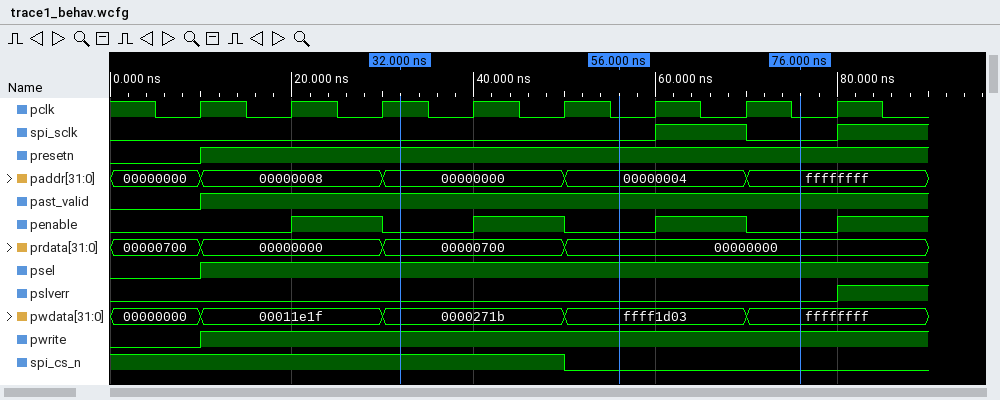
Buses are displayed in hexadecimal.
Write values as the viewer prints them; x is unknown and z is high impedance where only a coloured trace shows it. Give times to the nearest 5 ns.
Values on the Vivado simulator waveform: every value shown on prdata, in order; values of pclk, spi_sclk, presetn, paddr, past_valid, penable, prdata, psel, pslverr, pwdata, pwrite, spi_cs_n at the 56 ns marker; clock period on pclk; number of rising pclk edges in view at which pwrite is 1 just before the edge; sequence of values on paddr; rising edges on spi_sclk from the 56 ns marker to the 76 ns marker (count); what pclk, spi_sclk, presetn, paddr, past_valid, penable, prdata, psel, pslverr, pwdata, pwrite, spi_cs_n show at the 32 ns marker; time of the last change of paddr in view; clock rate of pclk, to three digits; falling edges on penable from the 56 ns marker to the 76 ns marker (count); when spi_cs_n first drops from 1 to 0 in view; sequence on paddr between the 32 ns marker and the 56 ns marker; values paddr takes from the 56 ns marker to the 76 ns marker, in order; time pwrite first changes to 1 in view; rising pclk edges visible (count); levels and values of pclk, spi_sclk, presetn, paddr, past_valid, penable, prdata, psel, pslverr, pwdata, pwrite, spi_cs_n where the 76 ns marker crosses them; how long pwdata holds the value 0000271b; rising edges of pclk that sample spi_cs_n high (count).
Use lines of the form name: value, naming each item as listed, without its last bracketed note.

every value shown on prdata, in order: 00000700, 00000000, 00000700, 00000000
values of pclk, spi_sclk, presetn, paddr, past_valid, penable, prdata, psel, pslverr, pwdata, pwrite, spi_cs_n at the 56 ns marker: pclk=0, spi_sclk=0, presetn=1, paddr=00000004, past_valid=1, penable=0, prdata=00000000, psel=1, pslverr=0, pwdata=ffff1d03, pwrite=1, spi_cs_n=0
clock period on pclk: 10 ns
number of rising pclk edges in view at which pwrite is 1 just before the edge: 7
sequence of values on paddr: 00000000, 00000008, 00000000, 00000004, ffffffff
rising edges on spi_sclk from the 56 ns marker to the 76 ns marker: 1
what pclk, spi_sclk, presetn, paddr, past_valid, penable, prdata, psel, pslverr, pwdata, pwrite, spi_cs_n show at the 32 ns marker: pclk=1, spi_sclk=0, presetn=1, paddr=00000000, past_valid=1, penable=0, prdata=00000700, psel=1, pslverr=0, pwdata=0000271b, pwrite=1, spi_cs_n=1
time of the last change of paddr in view: 70 ns
clock rate of pclk, to three digits: 100 MHz
falling edges on penable from the 56 ns marker to the 76 ns marker: 1
when spi_cs_n first drops from 1 to 0 in view: 50 ns
sequence on paddr between the 32 ns marker and the 56 ns marker: 00000000, 00000004
values paddr takes from the 56 ns marker to the 76 ns marker, in order: 00000004, ffffffff
time pwrite first changes to 1 in view: 10 ns
rising pclk edges visible: 8
levels and values of pclk, spi_sclk, presetn, paddr, past_valid, penable, prdata, psel, pslverr, pwdata, pwrite, spi_cs_n where the 76 ns marker crosses them: pclk=0, spi_sclk=0, presetn=1, paddr=ffffffff, past_valid=1, penable=0, prdata=00000000, psel=1, pslverr=0, pwdata=ffffffff, pwrite=1, spi_cs_n=0
how long pwdata holds the value 0000271b: 20 ns
rising edges of pclk that sample spi_cs_n high: 5
